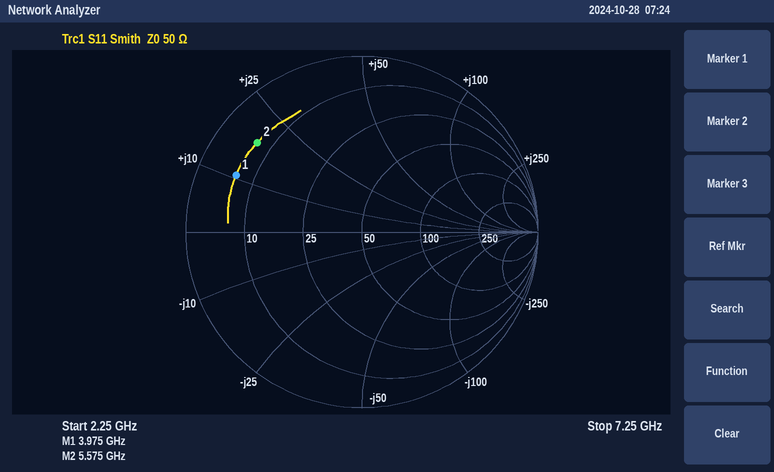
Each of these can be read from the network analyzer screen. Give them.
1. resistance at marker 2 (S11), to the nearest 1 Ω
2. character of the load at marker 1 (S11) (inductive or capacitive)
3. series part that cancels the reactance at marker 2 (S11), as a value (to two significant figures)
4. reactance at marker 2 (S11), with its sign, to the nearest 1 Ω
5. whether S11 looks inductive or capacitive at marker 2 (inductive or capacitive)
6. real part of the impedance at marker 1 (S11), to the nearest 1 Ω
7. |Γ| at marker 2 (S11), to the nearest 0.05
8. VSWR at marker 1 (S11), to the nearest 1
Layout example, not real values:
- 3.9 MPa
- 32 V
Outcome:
- 7 Ω
- inductive
- 1.6 pF
- +18 Ω
- inductive
- 6 Ω
- 0.80
- 8
